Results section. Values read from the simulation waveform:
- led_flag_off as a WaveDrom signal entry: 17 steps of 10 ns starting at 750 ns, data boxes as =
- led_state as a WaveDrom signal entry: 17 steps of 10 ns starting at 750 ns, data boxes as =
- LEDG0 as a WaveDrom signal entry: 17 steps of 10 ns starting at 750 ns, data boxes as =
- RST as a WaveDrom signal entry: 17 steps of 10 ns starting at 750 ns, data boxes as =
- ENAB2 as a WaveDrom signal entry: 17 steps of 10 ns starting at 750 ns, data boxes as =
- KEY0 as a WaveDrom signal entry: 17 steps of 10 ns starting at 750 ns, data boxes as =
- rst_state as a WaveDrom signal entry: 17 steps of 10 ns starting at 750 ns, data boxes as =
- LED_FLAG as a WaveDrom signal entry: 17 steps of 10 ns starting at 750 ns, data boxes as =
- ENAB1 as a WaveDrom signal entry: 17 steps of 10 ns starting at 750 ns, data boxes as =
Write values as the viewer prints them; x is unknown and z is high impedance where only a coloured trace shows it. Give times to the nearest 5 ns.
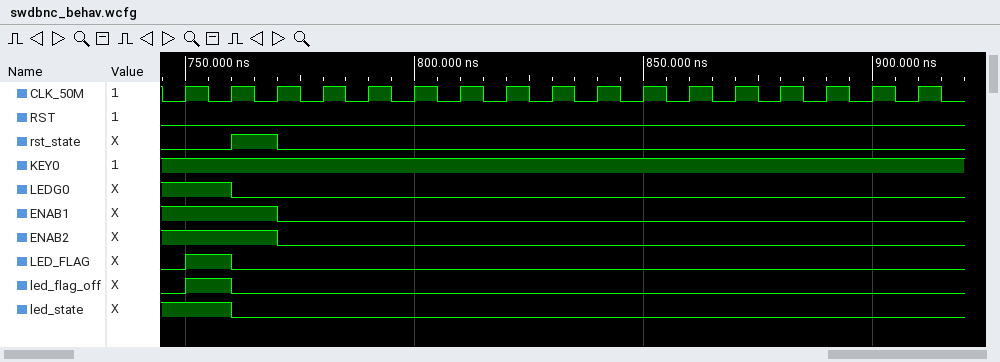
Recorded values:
{name: 'led_flag_off', wave: '10...............'}
{name: 'led_state', wave: '10...............'}
{name: 'LEDG0', wave: '10...............'}
{name: 'RST', wave: '0................'}
{name: 'ENAB2', wave: '1.0..............'}
{name: 'KEY0', wave: '1................'}
{name: 'rst_state', wave: '010..............'}
{name: 'LED_FLAG', wave: '10...............'}
{name: 'ENAB1', wave: '1.0..............'}
